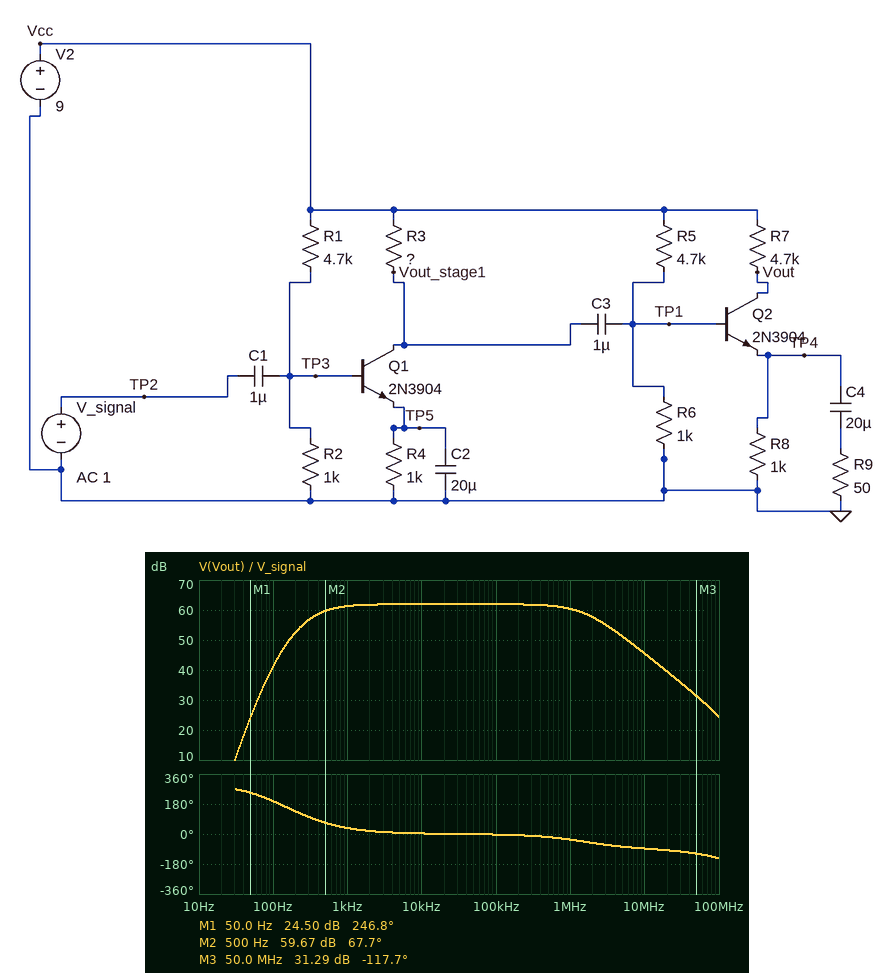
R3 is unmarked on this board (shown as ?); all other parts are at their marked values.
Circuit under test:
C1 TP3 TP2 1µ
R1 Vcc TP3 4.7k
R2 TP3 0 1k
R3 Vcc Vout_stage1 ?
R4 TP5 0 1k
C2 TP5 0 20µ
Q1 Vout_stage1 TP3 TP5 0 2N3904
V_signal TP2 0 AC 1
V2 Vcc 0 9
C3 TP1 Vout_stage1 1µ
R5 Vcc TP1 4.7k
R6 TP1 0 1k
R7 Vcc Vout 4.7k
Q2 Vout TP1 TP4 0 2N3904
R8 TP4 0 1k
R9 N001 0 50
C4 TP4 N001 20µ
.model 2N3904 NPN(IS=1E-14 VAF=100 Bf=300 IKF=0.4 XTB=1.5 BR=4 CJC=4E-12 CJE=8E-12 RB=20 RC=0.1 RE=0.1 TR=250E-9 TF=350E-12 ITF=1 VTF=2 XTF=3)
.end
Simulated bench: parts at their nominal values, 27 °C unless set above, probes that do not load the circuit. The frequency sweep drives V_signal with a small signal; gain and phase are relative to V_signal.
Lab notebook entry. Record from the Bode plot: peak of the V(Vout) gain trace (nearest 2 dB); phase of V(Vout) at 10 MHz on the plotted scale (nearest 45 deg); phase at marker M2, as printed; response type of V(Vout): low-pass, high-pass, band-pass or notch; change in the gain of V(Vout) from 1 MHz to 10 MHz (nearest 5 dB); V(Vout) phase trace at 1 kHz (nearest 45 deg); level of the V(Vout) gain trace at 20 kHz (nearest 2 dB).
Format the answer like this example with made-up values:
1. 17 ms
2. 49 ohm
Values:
1. 62 dB
2. -90 deg
3. 67.7 deg
4. band-pass
5. -15 dB
6. 45 deg
7. 62 dB
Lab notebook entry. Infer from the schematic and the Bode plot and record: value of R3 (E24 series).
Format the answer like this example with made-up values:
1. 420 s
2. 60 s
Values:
1. 2.2 kΩ
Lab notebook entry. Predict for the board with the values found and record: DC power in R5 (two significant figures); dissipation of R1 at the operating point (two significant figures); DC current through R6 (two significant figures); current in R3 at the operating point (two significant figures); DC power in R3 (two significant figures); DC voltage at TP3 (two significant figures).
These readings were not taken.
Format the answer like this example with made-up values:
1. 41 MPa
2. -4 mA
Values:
1. 12 mW
2. 12 mW
3. 1.6 mA
4. 920 µA
5. 1.9 mW
6. 1.6 V
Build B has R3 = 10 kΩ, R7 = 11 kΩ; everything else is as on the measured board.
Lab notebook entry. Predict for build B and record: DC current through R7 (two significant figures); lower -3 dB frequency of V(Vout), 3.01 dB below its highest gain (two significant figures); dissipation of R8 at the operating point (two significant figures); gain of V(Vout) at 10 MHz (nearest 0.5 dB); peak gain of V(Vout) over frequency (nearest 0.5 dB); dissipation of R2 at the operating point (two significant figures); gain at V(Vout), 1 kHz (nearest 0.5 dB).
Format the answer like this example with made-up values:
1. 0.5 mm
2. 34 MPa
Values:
1. 740 µA
2. 1.5 kHz
3. 700 µW
4. -8.5 dB
5. 0.5 dB
6. 2.3 mW
7. -5.5 dB
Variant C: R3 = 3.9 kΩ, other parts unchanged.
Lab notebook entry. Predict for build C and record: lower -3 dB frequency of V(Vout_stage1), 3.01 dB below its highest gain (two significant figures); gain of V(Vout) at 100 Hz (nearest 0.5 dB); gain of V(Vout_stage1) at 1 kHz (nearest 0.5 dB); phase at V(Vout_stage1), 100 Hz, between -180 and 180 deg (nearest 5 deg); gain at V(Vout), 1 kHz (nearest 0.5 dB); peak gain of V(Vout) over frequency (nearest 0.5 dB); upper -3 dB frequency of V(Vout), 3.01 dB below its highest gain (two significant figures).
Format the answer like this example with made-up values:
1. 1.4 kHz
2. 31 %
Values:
1. 300 Hz
2. 43.0 dB
3. 27.0 dB
4. -95 deg
5. 62.5 dB
6. 63.0 dB
7. 1.4 MHz
